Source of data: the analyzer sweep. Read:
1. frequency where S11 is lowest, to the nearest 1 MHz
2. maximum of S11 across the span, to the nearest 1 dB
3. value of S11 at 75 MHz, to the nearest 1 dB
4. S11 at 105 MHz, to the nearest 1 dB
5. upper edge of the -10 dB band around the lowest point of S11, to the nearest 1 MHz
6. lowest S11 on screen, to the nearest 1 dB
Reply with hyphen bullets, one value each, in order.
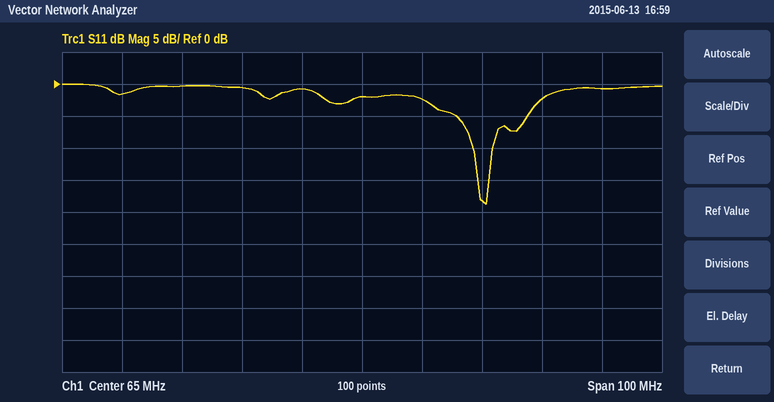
- 86 MHz
- 0 dB
- -2 dB
- -1 dB
- 87 MHz
- -19 dB
